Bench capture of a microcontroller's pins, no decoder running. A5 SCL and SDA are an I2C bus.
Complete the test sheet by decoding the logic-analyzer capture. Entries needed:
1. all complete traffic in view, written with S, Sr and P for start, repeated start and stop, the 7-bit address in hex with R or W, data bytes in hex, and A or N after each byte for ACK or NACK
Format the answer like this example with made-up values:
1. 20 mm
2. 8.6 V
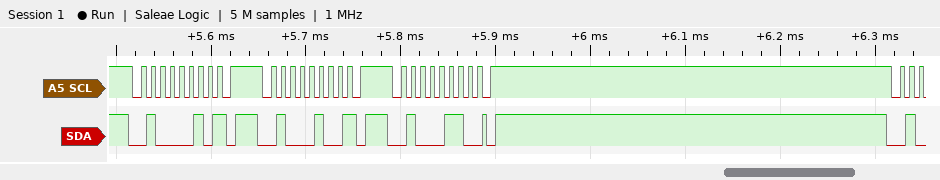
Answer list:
1. S 21W N P S 22W N P S 23W A P
